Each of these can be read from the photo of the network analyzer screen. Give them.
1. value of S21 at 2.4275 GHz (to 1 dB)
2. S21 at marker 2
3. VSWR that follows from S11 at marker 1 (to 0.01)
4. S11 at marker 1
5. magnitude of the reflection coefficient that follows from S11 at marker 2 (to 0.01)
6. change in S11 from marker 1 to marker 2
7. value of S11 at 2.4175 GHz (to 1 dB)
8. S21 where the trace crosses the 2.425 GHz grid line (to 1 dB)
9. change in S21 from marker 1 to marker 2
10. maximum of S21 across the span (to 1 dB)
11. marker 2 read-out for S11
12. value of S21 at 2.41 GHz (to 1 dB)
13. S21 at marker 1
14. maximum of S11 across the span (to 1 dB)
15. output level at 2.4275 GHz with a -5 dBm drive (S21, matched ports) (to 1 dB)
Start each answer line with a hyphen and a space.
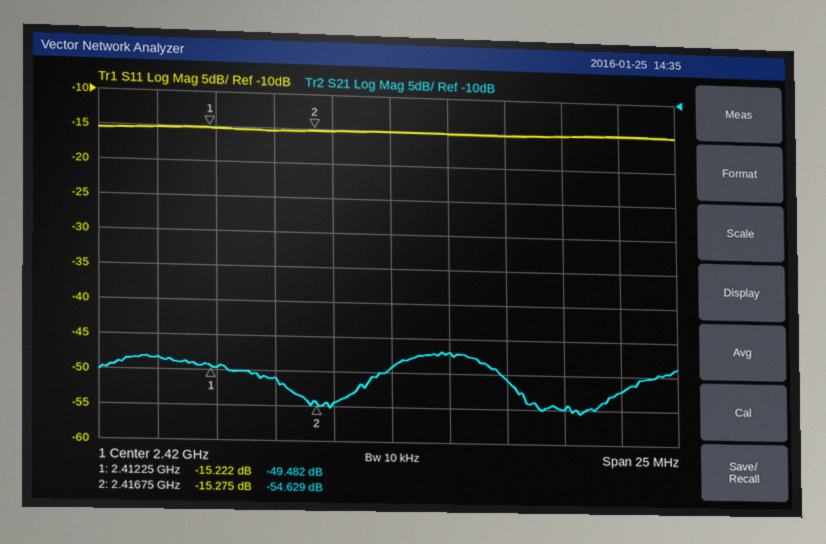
- -55 dB
- -54.629 dB
- 1.42
- -15.222 dB
- 0.17
- -0.053 dB
- -15 dB
- -51 dB
- -5.147 dB
- -47 dB
- -15.275 dB
- -48 dB
- -49.482 dB
- -15 dB
- -60 dBm
